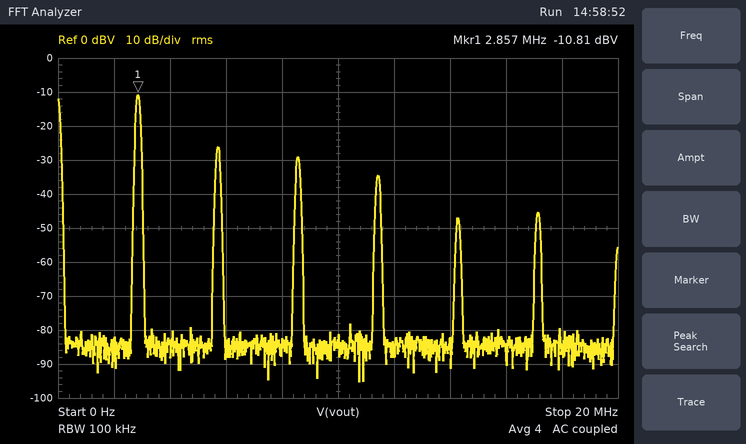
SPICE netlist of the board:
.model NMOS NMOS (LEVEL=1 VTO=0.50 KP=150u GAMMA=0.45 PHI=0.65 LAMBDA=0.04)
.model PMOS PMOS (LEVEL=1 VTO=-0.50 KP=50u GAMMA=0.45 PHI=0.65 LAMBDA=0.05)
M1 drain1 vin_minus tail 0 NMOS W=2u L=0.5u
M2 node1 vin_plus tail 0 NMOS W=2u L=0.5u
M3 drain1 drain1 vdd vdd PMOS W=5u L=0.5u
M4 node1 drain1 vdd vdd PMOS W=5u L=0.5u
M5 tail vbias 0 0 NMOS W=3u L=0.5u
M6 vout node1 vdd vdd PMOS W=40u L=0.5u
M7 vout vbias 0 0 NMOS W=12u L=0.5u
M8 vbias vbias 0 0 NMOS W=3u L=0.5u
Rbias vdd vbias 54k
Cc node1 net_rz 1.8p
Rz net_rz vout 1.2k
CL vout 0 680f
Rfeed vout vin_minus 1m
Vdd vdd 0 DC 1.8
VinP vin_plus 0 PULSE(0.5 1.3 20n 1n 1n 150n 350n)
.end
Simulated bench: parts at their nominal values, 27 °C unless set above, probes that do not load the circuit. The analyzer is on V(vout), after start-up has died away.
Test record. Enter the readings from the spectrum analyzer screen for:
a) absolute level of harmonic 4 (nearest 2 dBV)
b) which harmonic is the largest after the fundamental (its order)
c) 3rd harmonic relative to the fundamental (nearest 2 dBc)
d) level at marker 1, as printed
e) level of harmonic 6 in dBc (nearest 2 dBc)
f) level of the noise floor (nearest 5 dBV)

-34 dBV
2
-18 dBc
-10.81 dBV
-34 dBc
-85 dBV
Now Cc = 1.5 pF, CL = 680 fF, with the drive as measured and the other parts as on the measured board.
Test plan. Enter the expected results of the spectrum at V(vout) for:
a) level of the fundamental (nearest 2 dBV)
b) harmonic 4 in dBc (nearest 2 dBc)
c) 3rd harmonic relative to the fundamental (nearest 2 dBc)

-10 dBV
-22 dBc
-16 dBc
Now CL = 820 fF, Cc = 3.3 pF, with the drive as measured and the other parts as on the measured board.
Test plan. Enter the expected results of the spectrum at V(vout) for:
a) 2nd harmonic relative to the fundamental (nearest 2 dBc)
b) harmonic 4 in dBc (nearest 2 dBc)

-18 dBc
-32 dBc
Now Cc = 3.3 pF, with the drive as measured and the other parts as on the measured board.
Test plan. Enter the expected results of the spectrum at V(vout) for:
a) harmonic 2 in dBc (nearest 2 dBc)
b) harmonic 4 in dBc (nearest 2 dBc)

-18 dBc
-32 dBc
